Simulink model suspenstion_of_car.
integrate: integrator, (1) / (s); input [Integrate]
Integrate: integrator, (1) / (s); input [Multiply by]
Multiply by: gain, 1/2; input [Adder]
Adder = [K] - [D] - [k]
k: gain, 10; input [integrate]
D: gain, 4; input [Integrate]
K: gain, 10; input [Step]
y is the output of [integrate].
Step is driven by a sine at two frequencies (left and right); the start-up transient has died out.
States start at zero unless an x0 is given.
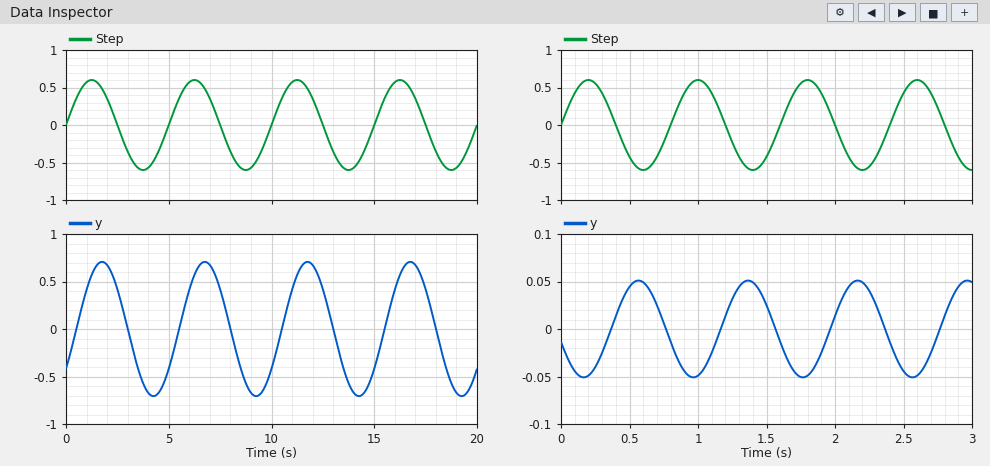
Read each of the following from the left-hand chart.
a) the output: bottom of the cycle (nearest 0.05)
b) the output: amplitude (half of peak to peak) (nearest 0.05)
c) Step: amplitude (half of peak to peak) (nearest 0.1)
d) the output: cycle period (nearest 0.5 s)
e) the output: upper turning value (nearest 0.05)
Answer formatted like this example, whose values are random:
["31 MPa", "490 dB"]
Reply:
["-0.70", "0.70", "0.6", "5.0 s", "0.70"]
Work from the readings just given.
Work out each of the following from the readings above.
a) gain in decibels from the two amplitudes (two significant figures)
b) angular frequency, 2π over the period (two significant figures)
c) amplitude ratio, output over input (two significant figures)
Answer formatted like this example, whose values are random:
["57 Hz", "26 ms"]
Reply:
["1.3 dB", "1.3 rad/s", "1.2"]
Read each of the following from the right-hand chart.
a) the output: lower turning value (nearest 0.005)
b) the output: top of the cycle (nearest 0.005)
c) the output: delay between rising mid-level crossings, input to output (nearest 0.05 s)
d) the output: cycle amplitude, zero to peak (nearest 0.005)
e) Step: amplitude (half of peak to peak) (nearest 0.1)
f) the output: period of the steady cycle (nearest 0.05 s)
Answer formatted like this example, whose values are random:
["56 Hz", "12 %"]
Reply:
["-0.050", "0.050", "0.35 s", "0.050", "0.6", "0.80 s"]
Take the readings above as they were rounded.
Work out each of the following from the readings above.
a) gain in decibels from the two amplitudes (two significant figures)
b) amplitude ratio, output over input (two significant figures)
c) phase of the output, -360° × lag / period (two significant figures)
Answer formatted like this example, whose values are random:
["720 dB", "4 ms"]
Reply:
["-22 dB", "0.083", "-160°"]
